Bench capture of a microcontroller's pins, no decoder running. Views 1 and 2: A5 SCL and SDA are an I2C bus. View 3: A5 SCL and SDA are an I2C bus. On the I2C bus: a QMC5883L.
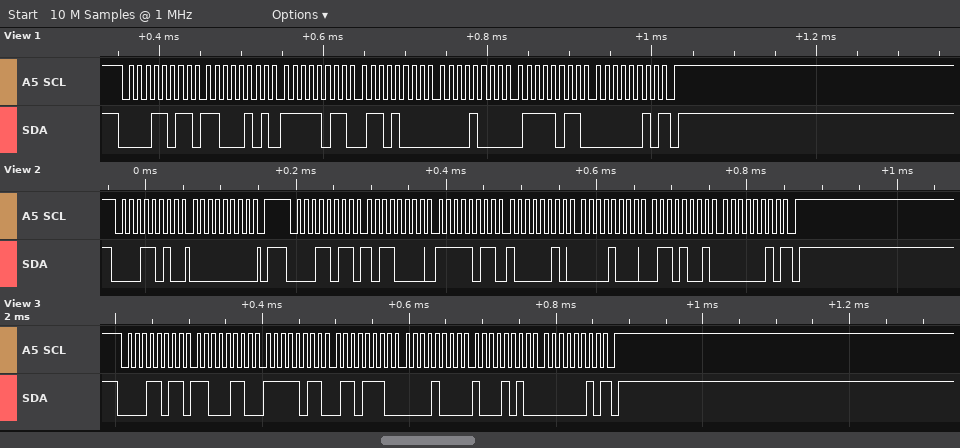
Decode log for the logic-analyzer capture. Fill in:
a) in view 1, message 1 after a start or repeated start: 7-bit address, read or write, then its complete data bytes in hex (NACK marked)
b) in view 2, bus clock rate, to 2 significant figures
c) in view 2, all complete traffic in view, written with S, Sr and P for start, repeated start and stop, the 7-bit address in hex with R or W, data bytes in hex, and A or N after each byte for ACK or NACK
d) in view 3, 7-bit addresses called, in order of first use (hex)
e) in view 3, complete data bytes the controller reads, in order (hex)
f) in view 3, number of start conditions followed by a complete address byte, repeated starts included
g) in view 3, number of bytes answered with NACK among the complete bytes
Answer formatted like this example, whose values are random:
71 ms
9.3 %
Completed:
0x0D read: C5 FB 68 08 7B 02 NACK
100 kHz
S 0DW A 00 A P S 0DR A B0 A FB A 82 A 08 A 69 A 02 N P
0x0D
C6 FB 6E 08 8A 02
1
1
